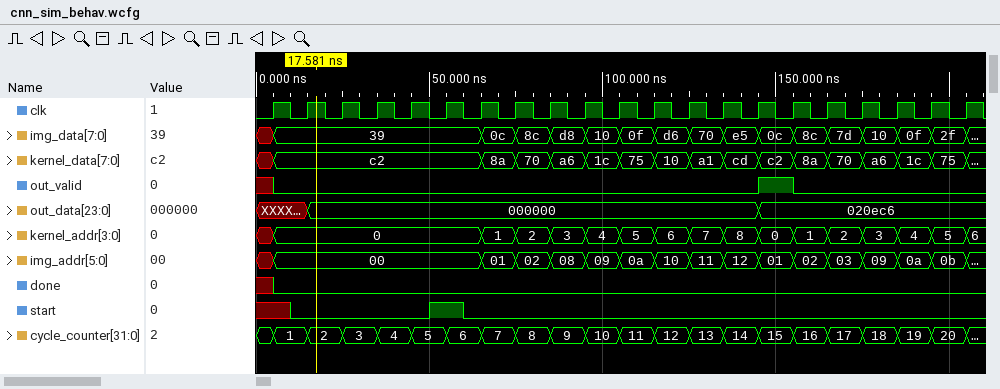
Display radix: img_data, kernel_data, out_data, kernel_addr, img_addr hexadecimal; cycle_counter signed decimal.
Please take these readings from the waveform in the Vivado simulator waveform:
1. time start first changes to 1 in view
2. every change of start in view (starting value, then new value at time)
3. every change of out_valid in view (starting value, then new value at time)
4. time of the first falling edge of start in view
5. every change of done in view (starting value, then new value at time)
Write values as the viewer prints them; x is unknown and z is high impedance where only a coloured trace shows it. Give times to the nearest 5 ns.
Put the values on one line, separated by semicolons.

50 ns; x, 0 at 10 ns, 1 at 50 ns, 0 at 60 ns; x, 0 at 5 ns, 1 at 145 ns, 0 at 155 ns; 60 ns; x, 0 at 5 ns
